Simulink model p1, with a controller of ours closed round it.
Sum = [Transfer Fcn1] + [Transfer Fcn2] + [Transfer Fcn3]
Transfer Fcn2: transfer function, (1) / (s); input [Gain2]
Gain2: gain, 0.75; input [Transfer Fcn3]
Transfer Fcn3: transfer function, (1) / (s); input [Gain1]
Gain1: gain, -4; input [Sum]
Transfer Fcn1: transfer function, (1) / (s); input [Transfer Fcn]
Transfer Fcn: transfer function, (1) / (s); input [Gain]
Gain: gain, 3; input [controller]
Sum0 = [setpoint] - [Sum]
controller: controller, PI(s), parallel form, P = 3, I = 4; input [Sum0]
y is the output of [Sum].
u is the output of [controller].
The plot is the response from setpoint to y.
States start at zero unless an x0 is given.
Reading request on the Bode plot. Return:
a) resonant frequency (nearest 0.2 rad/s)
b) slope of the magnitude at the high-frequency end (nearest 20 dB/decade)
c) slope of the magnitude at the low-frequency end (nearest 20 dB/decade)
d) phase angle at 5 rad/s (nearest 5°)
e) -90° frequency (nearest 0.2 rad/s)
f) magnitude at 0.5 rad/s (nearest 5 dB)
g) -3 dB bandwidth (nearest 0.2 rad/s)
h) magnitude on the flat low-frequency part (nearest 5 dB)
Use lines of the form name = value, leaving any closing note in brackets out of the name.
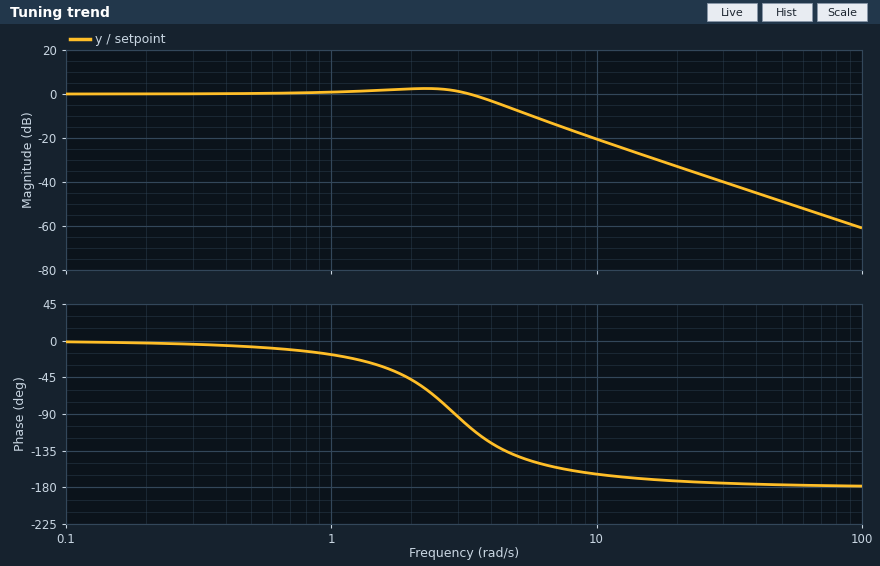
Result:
resonant frequency = 2.2 rad/s
slope of the magnitude at the high-frequency end = -40 dB/decade
slope of the magnitude at the low-frequency end = 0 dB/decade
phase angle at 5 rad/s = -140°
-90° frequency = 3.0 rad/s
magnitude at 0.5 rad/s = 0 dB
-3 dB bandwidth = 4.0 rad/s
magnitude on the flat low-frequency part = 0 dB
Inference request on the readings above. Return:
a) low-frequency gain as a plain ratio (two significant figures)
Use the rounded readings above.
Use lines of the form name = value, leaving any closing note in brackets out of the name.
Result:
low-frequency gain as a plain ratio = 1.0
